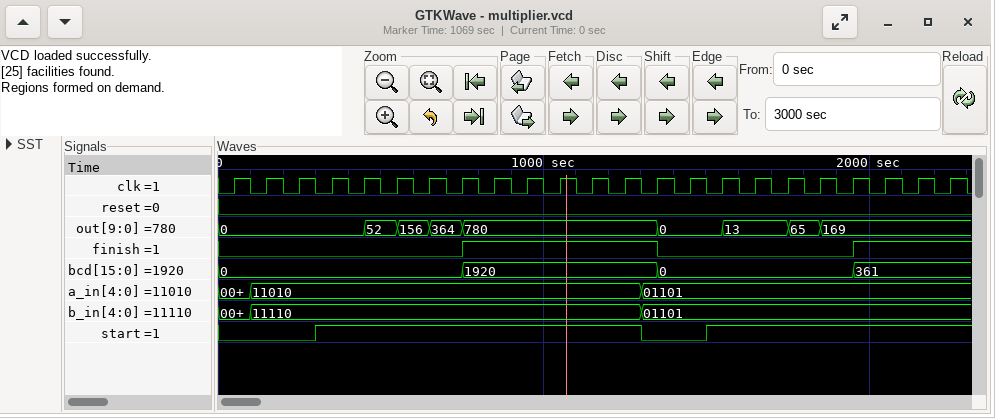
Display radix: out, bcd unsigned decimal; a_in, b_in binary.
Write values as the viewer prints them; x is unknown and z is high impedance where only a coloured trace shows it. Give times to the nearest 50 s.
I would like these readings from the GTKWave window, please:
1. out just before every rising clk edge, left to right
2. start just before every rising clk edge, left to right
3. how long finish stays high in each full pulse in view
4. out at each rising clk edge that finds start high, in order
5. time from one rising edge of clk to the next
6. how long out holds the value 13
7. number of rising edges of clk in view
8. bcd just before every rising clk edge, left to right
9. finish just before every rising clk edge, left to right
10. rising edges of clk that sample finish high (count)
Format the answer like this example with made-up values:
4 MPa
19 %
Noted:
0, 0, 0, 0, 0, 52, 156, 364, 780, 780, 780, 780, 780, 780, 0, 0, 13, 13, 65, 169, 169, 169, 169
0 0 0 1 1 1 1 1 1 1 1 1 1 0 0 1 1 1 1 1 1 1 1
600 s
0, 0, 52, 156, 364, 780, 780, 780, 780, 780, 0, 13, 13, 65, 169, 169, 169, 169
100 s
200 s
23
0, 0, 0, 0, 0, 0, 0, 0, 1920, 1920, 1920, 1920, 1920, 1920, 0, 0, 0, 0, 0, 0, 361, 361, 361
0 0 0 0 0 0 0 0 1 1 1 1 1 1 0 0 0 0 0 0 1 1 1
9
